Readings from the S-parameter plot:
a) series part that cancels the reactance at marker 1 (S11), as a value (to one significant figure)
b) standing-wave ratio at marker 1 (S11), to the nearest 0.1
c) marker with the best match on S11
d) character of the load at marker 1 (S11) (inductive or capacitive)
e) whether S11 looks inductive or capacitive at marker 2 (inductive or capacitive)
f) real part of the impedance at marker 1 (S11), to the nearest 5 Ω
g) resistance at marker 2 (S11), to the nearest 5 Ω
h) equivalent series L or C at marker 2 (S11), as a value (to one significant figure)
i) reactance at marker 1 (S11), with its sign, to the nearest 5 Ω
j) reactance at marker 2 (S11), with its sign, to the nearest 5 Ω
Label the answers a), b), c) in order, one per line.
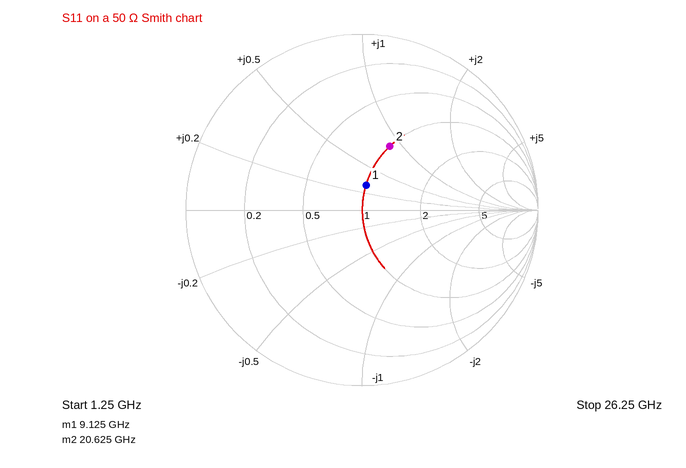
a) 1 pF
b) 1.3
c) marker 1
d) inductive
e) inductive
f) 50 Ω
g) 50 Ω
h) 300 pH
i) +15 Ω
j) +45 Ω
